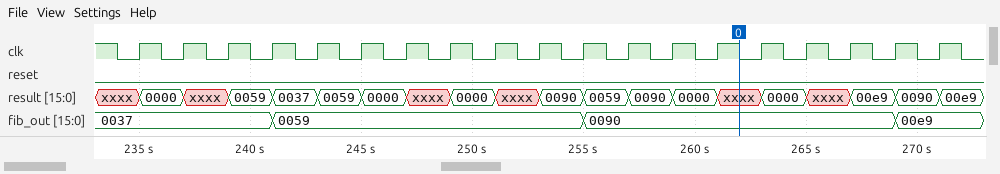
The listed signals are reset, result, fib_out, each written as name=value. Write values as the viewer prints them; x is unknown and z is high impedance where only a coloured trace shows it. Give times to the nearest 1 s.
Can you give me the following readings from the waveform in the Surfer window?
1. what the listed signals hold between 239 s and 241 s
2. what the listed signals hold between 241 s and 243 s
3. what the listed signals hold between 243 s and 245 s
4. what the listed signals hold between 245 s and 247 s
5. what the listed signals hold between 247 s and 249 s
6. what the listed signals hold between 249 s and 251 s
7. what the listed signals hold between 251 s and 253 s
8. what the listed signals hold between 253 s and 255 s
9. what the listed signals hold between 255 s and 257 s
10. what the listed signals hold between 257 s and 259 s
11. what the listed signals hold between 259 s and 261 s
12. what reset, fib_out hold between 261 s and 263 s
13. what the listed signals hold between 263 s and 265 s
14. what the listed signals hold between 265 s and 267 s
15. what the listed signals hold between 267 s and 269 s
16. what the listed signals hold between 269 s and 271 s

reset=0, result=0059, fib_out=0037
reset=0, result=0037, fib_out=0059
reset=0, result=0059, fib_out=0059
reset=0, result=0000, fib_out=0059
reset=0, result=xxxx, fib_out=0059
reset=0, result=0000, fib_out=0059
reset=0, result=xxxx, fib_out=0059
reset=0, result=0090, fib_out=0059
reset=0, result=0059, fib_out=0090
reset=0, result=0090, fib_out=0090
reset=0, result=0000, fib_out=0090
reset=0, fib_out=0090
reset=0, result=0000, fib_out=0090
reset=0, result=xxxx, fib_out=0090
reset=0, result=00e9, fib_out=0090
reset=0, result=0090, fib_out=00e9
